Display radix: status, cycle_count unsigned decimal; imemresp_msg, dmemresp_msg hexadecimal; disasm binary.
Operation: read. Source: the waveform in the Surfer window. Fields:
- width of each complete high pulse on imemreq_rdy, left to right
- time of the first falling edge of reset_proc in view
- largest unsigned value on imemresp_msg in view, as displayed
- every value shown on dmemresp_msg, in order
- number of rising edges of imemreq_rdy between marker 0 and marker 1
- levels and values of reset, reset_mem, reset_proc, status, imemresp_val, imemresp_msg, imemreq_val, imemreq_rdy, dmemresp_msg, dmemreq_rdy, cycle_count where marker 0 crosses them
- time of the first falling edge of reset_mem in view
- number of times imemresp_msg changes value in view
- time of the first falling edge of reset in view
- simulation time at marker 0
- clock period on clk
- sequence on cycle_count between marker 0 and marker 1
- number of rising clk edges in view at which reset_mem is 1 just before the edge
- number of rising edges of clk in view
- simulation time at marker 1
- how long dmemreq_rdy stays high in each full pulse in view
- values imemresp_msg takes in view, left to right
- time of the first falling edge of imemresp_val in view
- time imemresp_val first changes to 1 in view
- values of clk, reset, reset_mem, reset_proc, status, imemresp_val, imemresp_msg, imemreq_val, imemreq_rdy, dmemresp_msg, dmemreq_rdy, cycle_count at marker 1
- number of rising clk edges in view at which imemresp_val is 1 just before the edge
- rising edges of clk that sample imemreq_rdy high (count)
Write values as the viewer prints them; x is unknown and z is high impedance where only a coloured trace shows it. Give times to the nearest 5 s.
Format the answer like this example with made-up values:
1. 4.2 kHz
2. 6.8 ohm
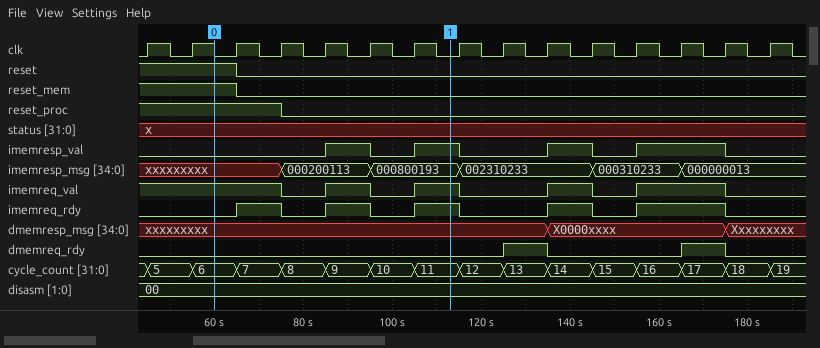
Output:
1. 10 s, 10 s, 10 s, 10 s, 20 s
2. 75 s
3. 002310233
4. xxxxxxxxx, X0000xxxx, Xxxxxxxxx
5. 3
6. reset=1, reset_mem=1, reset_proc=1, status=x, imemresp_val=0, imemresp_msg=xxxxxxxxx, imemreq_val=1, imemreq_rdy=0, dmemresp_msg=xxxxxxxxx, dmemreq_rdy=0, cycle_count=6
7. 65 s
8. 5
9. 65 s
10. 60 s
11. 10 s
12. 6, 7, 8, 9, 10, 11
13. 3
14. 15
15. 115 s
16. 10 s, 10 s
17. xxxxxxxxx, 000200113, 000800193, 002310233, 000310233, 000000013
18. 95 s
19. 85 s
20. clk=0, reset=0, reset_mem=0, reset_proc=0, status=x, imemresp_val=1, imemresp_msg=000800193, imemreq_val=1, imemreq_rdy=1, dmemresp_msg=xxxxxxxxx, dmemreq_rdy=0, cycle_count=11
21. 5
22. 6
